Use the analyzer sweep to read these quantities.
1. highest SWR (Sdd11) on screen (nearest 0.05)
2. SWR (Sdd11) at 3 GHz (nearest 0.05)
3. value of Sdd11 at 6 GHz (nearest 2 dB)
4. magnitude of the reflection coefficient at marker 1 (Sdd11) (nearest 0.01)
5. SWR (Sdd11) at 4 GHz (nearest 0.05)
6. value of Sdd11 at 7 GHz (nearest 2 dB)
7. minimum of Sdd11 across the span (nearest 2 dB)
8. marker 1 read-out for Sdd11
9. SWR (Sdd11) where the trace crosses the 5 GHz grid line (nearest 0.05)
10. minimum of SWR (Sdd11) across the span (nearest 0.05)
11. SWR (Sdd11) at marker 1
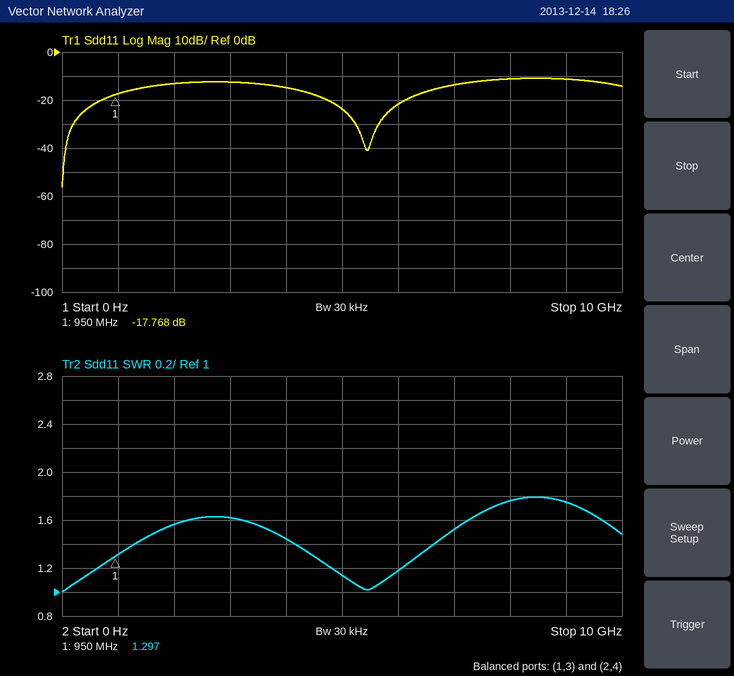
1.80
1.60
-22 dB
0.13
1.45
-14 dB
-56 dB
-17.768 dB
1.15
1.00
1.297
